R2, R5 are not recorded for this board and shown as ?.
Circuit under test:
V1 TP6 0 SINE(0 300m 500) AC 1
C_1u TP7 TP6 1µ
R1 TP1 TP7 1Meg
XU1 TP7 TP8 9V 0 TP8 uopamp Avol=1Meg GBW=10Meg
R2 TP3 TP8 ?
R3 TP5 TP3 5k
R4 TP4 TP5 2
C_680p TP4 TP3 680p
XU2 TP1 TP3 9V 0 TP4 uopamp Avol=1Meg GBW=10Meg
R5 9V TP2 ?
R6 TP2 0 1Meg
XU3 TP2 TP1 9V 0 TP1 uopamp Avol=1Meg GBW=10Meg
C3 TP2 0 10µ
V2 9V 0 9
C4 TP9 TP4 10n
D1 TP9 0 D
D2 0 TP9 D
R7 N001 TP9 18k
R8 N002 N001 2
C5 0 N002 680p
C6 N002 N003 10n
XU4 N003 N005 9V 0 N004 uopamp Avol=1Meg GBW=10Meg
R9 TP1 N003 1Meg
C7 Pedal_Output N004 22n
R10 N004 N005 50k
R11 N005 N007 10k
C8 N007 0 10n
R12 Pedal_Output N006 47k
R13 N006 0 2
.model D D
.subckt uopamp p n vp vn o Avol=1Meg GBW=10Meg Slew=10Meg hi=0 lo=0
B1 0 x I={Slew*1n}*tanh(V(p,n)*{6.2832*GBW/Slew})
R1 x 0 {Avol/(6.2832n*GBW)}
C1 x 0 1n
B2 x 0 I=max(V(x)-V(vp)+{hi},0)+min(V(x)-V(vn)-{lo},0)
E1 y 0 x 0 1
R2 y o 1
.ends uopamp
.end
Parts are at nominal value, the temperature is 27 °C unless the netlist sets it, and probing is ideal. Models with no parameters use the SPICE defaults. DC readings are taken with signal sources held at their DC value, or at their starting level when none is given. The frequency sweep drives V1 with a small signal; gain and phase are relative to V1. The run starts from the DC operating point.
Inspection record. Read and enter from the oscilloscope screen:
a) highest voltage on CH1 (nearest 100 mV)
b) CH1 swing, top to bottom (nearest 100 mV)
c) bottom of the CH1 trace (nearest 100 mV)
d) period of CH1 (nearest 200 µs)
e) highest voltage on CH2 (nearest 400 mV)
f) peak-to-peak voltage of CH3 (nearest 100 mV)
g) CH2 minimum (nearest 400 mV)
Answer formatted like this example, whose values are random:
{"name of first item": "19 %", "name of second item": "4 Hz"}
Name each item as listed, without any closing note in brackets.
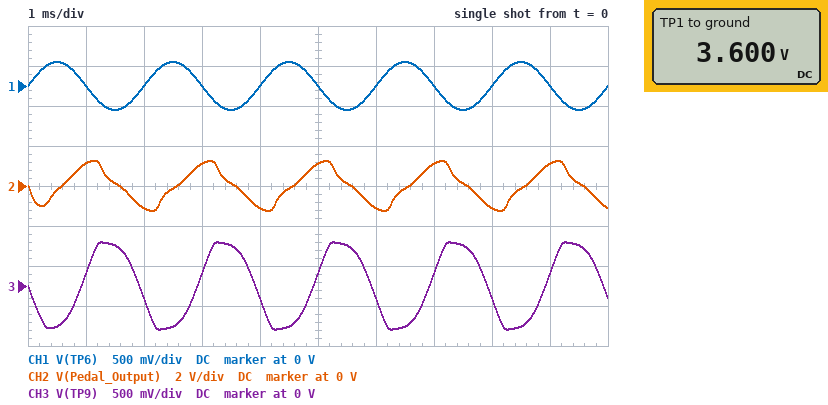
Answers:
{"highest voltage on CH1": "300 mV", "CH1 swing, top to bottom": "600 mV", "bottom of the CH1 trace": "-300 mV", "period of CH1": "2.0 ms", "highest voltage on CH2": "1.2 V", "peak-to-peak voltage of CH3": "1.1 V", "CH2 minimum": "-1.2 V"}
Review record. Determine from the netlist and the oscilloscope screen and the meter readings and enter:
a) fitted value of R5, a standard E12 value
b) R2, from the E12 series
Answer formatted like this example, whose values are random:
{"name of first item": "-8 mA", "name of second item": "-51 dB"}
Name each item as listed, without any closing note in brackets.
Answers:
{"fitted value of R5, a standard E12 value": "1.5 MΩ", "R2, from the E12 series": "2.2 kΩ"}
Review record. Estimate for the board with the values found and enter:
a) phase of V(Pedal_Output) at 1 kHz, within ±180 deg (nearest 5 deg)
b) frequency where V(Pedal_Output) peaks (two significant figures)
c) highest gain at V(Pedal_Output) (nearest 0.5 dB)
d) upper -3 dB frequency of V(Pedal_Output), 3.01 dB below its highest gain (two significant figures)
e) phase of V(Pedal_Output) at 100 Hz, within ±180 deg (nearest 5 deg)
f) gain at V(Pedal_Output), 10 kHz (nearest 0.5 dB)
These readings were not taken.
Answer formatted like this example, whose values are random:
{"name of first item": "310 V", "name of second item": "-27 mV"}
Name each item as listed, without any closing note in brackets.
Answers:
{"phase of V(Pedal_Output) at 1 kHz, within ±180 deg": "-130 deg", "frequency where V(Pedal_Output) peaks": "4.6 kHz", "highest gain at V(Pedal_Output)": "21.0 dB", "upper -3 dB frequency of V(Pedal_Output), 3.01 dB below its highest gain": "16 kHz", "phase of V(Pedal_Output) at 100 Hz, within ±180 deg": "-90 deg", "gain at V(Pedal_Output), 10 kHz": "20.0 dB"}
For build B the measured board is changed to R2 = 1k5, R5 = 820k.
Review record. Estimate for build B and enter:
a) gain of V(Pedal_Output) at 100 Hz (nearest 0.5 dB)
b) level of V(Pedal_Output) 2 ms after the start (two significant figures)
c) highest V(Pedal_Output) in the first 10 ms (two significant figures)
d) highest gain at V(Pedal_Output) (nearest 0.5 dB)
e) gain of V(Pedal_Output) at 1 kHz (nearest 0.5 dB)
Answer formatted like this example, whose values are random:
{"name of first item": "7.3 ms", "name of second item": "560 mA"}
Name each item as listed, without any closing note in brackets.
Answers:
{"gain of V(Pedal_Output) at 100 Hz": "4.5 dB", "level of V(Pedal_Output) 2 ms after the start": "-1.7 V", "highest V(Pedal_Output) in the first 10 ms": "1.7 V", "highest gain at V(Pedal_Output)": "24.5 dB", "gain of V(Pedal_Output) at 1 kHz": "20.0 dB"}
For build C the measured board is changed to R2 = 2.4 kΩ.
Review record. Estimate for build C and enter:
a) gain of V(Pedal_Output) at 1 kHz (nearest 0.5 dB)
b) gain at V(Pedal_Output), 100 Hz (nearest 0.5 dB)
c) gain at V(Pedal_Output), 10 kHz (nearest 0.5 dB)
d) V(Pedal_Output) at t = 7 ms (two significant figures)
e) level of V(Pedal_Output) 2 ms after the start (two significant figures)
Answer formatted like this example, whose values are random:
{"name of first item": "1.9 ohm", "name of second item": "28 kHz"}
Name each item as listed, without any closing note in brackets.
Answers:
{"gain of V(Pedal_Output) at 1 kHz": "16.0 dB", "gain at V(Pedal_Output), 100 Hz": "0.5 dB", "gain at V(Pedal_Output), 10 kHz": "19.0 dB", "V(Pedal_Output) at t = 7 ms": "1.0 V", "level of V(Pedal_Output) 2 ms after the start": "-1.0 V"}
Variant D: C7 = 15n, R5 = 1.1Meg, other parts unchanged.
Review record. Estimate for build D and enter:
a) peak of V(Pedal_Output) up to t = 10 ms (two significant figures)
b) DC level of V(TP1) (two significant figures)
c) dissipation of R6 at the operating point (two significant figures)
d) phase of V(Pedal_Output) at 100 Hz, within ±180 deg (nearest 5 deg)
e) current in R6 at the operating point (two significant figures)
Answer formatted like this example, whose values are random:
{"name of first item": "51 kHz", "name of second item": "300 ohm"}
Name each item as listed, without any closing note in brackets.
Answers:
{"peak of V(Pedal_Output) up to t = 10 ms": "1.2 V", "DC level of V(TP1)": "4.3 V", "dissipation of R6 at the operating point": "18 µW", "phase of V(Pedal_Output) at 100 Hz, within ±180 deg": "-80 deg", "current in R6 at the operating point": "4.3 µA"}
